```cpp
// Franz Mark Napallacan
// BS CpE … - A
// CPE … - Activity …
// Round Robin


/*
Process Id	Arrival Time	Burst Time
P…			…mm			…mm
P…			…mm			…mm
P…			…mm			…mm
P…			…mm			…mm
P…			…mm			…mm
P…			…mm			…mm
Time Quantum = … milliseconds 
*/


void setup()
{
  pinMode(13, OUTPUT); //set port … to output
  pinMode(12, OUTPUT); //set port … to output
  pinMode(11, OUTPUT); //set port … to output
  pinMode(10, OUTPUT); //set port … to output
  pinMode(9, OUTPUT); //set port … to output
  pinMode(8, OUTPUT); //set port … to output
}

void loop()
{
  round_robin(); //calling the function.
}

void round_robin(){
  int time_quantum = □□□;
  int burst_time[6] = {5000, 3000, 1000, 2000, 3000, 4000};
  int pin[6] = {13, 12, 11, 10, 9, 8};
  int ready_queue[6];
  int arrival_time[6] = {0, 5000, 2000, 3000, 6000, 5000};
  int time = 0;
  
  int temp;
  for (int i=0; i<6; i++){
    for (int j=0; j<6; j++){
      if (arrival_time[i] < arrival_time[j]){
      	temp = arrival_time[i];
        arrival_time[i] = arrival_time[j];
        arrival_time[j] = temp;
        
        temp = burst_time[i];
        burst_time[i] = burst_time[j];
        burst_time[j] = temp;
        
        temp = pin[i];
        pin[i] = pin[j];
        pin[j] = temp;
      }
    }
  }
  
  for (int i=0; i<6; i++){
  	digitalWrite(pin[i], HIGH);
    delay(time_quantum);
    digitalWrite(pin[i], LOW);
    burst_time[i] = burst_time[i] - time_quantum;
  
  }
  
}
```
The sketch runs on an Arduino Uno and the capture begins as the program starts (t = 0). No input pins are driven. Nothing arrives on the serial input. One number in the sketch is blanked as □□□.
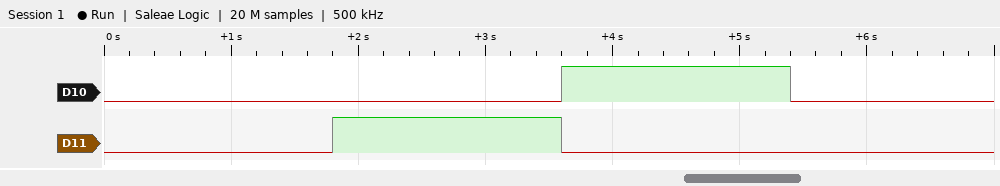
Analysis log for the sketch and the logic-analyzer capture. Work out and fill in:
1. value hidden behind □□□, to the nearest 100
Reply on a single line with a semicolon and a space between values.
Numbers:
1800
